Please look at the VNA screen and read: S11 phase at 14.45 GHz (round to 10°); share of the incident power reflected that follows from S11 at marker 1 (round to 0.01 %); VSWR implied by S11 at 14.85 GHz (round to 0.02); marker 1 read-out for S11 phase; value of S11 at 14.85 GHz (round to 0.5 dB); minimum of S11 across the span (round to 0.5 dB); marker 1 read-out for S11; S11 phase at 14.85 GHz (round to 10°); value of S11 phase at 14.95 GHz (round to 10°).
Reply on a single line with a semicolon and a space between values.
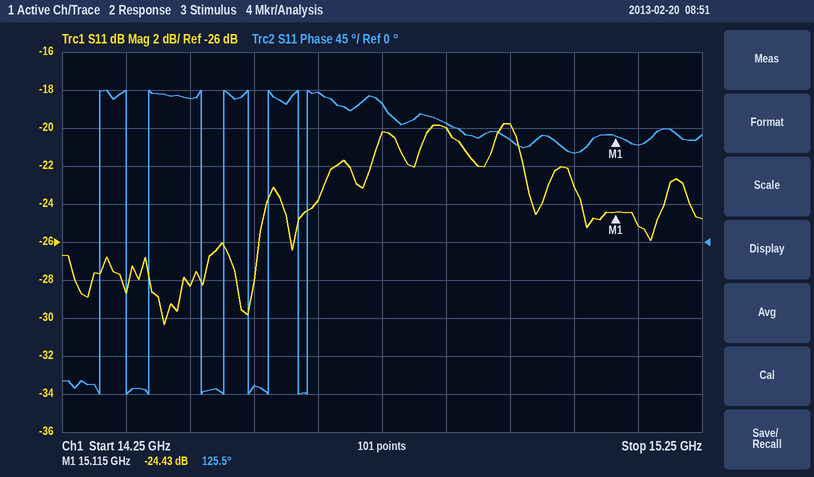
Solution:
170°; 0.36 %; 1.22; 125.5°; -20.0 dB; -30.5 dB; -24.43 dB; 140°; 120°
